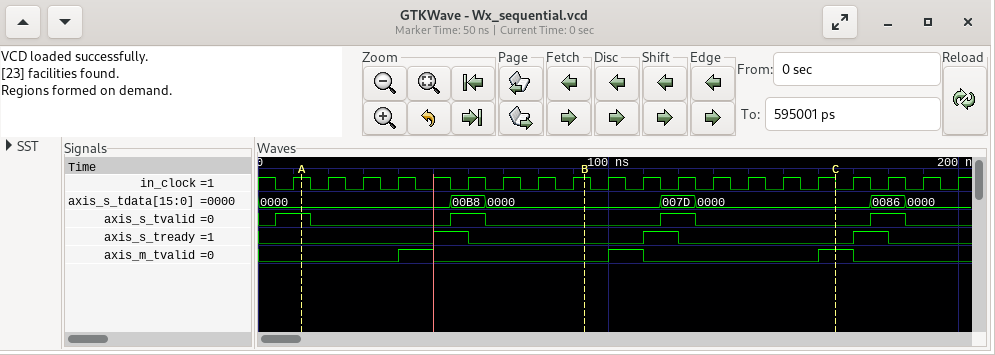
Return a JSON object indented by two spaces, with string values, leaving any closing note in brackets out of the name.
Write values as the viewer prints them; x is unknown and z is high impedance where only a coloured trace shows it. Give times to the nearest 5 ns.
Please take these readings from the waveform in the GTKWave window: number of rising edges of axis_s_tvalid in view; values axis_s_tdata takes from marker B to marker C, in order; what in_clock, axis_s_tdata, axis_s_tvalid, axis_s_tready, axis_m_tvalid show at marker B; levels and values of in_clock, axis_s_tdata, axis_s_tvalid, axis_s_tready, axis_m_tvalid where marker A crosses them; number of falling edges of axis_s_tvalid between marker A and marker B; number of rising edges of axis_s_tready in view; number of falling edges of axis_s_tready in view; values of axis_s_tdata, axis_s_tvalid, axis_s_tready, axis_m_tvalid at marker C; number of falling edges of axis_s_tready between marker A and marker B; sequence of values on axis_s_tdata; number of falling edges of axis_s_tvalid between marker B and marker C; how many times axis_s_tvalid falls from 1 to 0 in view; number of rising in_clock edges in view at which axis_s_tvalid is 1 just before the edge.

{
  "number of rising edges of axis_s_tvalid in view": "4",
  "values axis_s_tdata takes from marker B to marker C, in order": "0000, 007D, 0000",
  "what in_clock, axis_s_tdata, axis_s_tvalid, axis_s_tready, axis_m_tvalid show at marker B": "in_clock=1, axis_s_tdata=0000, axis_s_tvalid=0, axis_s_tready=0, axis_m_tvalid=0",
  "levels and values of in_clock, axis_s_tdata, axis_s_tvalid, axis_s_tready, axis_m_tvalid where marker A crosses them": "in_clock=1, axis_s_tdata=0000, axis_s_tvalid=1, axis_s_tready=0, axis_m_tvalid=0",
  "number of falling edges of axis_s_tvalid between marker A and marker B": "2",
  "number of rising edges of axis_s_tready in view": "3",
  "number of falling edges of axis_s_tready in view": "3",
  "values of axis_s_tdata, axis_s_tvalid, axis_s_tready, axis_m_tvalid at marker C": "axis_s_tdata=0000, axis_s_tvalid=0, axis_s_tready=0, axis_m_tvalid=1",
  "number of falling edges of axis_s_tready between marker A and marker B": "1",
  "sequence of values on axis_s_tdata": "0000, 00B8, 0000, 007D, 0000, 0086, 0000",
  "number of falling edges of axis_s_tvalid between marker B and marker C": "1",
  "how many times axis_s_tvalid falls from 1 to 0 in view": "4",
  "number of rising in_clock edges in view at which axis_s_tvalid is 1 just before the edge": "4"
}
